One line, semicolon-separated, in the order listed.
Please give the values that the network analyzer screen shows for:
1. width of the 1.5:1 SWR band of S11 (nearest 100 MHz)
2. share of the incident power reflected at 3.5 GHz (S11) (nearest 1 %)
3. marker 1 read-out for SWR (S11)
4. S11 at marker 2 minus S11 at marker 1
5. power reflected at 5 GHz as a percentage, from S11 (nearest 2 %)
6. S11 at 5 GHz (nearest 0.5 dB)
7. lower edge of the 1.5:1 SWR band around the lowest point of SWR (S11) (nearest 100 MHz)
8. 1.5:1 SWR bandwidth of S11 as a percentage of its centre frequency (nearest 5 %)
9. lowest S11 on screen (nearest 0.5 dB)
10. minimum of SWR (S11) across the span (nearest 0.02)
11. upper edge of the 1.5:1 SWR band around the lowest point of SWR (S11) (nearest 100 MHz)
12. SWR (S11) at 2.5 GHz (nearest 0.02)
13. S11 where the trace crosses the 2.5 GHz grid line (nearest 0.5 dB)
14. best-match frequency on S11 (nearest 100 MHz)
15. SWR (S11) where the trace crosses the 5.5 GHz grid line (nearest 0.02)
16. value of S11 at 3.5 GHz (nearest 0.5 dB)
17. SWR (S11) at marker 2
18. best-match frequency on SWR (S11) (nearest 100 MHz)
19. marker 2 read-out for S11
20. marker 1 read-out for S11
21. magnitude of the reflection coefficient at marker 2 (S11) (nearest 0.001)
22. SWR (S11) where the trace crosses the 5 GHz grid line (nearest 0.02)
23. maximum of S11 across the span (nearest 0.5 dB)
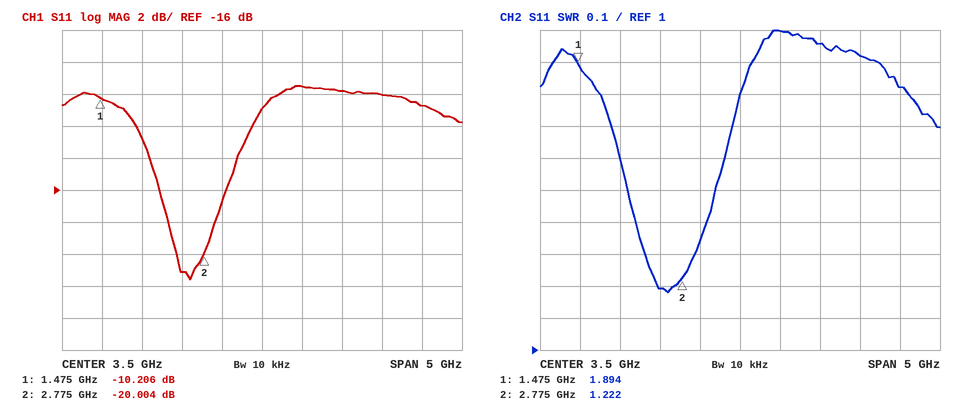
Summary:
1.1 GHz; 8 %; 1.894; -9.798 dB; 10 %; -10.0 dB; 2.1 GHz; 40 %; -21.5 dB; 1.18; 3.2 GHz; 1.20; -21.0 dB; 2.6 GHz; 1.82; -11.0 dB; 1.222; 2.6 GHz; -20.004 dB; -10.206 dB; 0.100; 1.92; -9.5 dB
